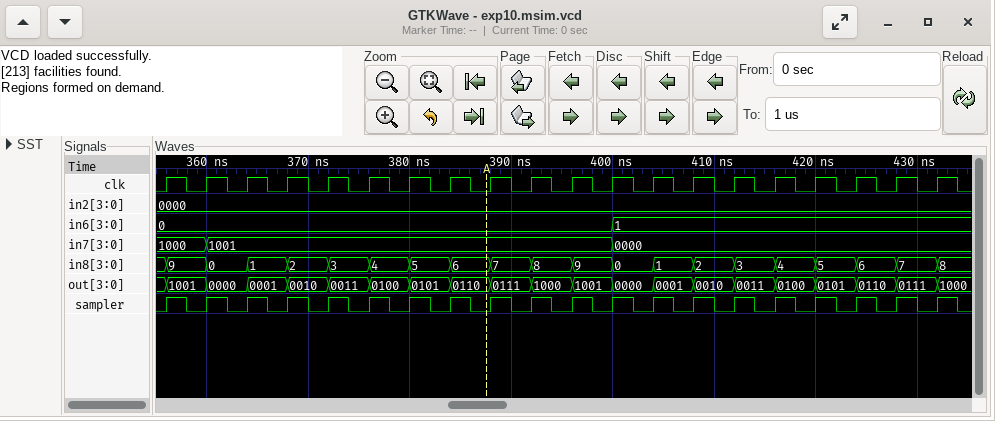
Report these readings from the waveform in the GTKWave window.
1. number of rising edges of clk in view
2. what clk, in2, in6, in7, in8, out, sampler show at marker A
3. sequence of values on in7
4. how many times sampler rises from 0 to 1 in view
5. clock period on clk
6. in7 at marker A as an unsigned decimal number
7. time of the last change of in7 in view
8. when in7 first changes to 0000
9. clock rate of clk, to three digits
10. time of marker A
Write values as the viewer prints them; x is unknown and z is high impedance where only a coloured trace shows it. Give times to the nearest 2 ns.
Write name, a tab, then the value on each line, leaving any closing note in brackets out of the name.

number of rising edges of clk in view	20
what clk, in2, in6, in7, in8, out, sampler show at marker A	clk=0, in2=0000, in6=0, in7=1001, in8=6, out=0110, sampler=0
sequence of values on in7	1000, 1001, 0000
how many times sampler rises from 0 to 1 in view	20
clock period on clk	4 ns
in7 at marker A as an unsigned decimal number	9
time of the last change of in7 in view	400 ns
when in7 first changes to 0000	400 ns
clock rate of clk, to three digits	250 MHz
time of marker A	388 ns
